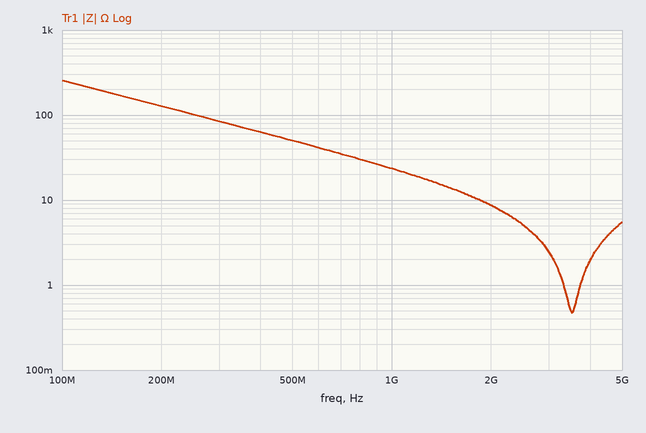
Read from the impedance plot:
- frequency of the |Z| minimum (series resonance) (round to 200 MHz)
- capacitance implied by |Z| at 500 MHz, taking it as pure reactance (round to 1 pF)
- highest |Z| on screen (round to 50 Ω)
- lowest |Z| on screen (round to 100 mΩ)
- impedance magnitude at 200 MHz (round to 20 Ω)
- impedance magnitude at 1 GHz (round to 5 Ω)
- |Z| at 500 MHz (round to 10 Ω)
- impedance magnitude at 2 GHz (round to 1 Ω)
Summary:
3.6 GHz
6 pF
250 Ω
500 mΩ
120 Ω
25 Ω
50 Ω
9 Ω
